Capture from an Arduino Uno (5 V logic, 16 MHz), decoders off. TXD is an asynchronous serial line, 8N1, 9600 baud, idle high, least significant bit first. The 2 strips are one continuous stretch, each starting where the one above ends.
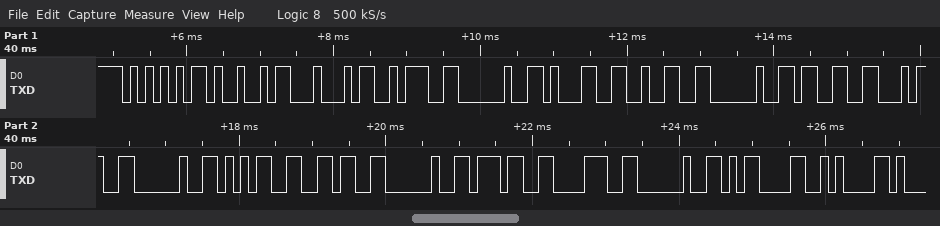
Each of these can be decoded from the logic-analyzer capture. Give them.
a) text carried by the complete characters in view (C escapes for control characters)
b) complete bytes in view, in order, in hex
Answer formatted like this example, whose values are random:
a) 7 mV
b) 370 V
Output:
a) "UID: 12 34 56 78 \r\n"
b) 55 49 44 3A 20 31 32 20 33 34 20 35 36 20 37 38 20 0D 0A
